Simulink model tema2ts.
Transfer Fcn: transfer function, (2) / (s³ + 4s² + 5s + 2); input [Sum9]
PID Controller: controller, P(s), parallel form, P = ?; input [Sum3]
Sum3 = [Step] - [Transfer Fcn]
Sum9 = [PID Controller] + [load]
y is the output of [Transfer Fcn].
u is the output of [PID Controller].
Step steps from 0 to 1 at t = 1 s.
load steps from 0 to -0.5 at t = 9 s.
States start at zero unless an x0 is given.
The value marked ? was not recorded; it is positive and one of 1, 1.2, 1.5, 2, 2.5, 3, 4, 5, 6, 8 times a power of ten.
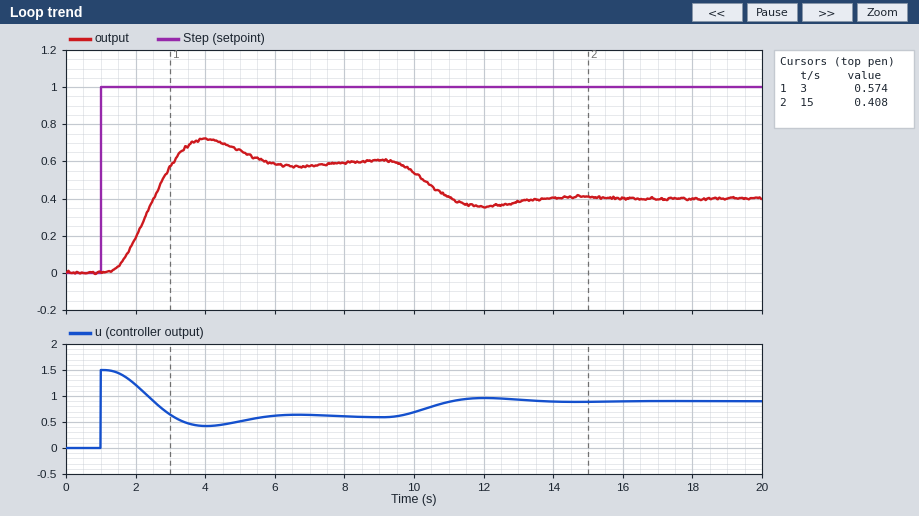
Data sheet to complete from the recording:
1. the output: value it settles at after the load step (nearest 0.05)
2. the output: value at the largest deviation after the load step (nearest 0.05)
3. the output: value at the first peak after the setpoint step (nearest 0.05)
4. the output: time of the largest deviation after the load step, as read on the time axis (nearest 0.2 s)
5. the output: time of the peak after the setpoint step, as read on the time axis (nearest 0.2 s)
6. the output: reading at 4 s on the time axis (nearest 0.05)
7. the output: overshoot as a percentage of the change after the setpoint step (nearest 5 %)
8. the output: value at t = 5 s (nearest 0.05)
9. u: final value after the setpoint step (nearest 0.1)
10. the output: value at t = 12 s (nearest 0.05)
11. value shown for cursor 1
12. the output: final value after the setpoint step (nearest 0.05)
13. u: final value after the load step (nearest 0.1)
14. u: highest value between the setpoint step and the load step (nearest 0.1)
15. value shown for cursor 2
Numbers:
0.40
0.35
0.70
12.0 s
4.0 s
0.70
20 %
0.65
0.6
0.35
0.574
0.60
0.9
1.5
0.408
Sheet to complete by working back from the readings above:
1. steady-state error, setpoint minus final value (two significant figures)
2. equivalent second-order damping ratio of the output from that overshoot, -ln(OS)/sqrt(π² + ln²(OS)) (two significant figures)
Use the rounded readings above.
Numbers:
0.40
0.46
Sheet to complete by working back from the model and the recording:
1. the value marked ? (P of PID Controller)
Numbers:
1.5
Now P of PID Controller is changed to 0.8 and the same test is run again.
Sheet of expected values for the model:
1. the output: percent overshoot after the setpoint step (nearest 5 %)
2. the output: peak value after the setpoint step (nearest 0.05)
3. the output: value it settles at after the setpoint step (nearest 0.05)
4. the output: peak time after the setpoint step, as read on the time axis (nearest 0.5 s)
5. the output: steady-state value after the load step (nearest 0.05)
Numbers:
10 %
0.50
0.45
5.0 s
0.15
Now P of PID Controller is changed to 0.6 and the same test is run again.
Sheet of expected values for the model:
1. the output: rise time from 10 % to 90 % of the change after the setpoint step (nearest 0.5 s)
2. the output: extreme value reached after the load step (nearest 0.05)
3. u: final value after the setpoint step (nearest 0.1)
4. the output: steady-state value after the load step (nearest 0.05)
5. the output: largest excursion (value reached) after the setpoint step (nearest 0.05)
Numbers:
2.0 s
0.05
0.4
0.05
0.40
